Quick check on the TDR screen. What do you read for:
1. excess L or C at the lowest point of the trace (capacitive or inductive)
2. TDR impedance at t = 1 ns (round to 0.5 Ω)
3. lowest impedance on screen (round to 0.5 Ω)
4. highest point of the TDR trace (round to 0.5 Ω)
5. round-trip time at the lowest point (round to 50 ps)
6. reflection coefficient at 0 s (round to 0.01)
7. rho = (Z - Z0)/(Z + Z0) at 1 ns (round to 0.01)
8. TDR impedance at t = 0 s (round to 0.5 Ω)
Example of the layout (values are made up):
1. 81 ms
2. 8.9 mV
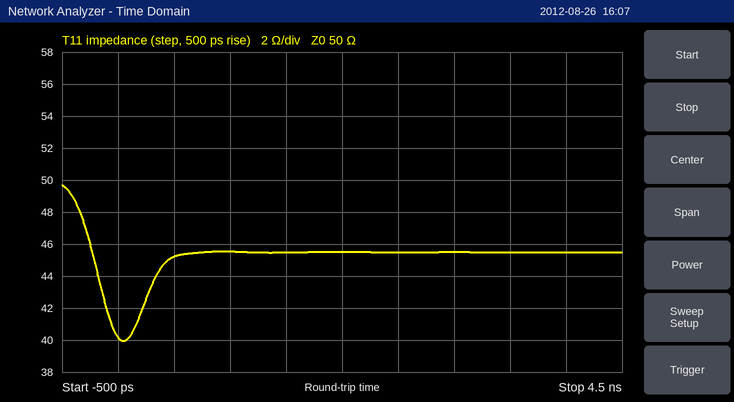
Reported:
1. capacitive
2. 45.5 Ω
3. 40.0 Ω
4. 49.5 Ω
5. 50 ps
6. -0.11
7. -0.05
8. 40.0 Ω
